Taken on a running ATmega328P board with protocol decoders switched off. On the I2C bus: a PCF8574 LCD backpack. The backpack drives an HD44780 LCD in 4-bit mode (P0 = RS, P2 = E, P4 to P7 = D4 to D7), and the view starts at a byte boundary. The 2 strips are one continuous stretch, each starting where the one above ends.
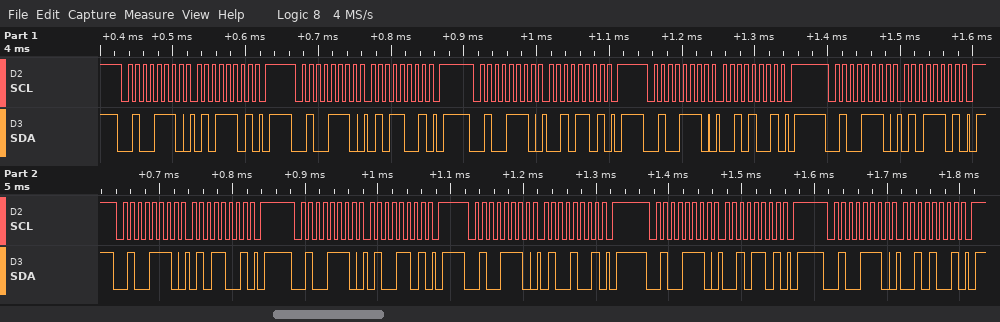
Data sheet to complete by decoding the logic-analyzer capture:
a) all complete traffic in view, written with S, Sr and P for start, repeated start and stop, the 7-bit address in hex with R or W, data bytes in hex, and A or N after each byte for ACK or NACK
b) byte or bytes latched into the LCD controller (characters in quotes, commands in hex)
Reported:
S 27W A 5D A P S 27W A 59 A P S 27W A 2D A P S 27W A 29 A P S 27W A 5D A P S 27W A 59 A P S 27W A 4D A P S 27W A 49 A P S 27W A 2D A P S 27W A 29 A P
'R' 'T'
